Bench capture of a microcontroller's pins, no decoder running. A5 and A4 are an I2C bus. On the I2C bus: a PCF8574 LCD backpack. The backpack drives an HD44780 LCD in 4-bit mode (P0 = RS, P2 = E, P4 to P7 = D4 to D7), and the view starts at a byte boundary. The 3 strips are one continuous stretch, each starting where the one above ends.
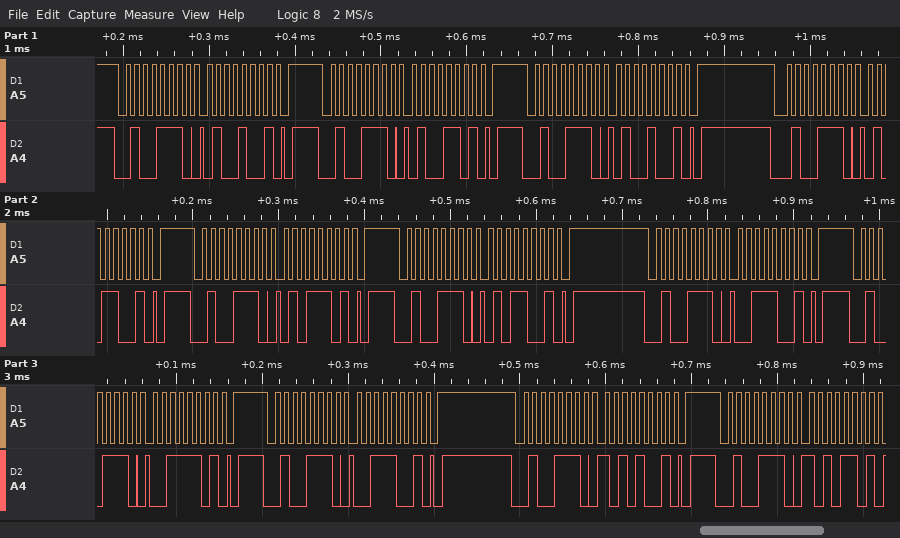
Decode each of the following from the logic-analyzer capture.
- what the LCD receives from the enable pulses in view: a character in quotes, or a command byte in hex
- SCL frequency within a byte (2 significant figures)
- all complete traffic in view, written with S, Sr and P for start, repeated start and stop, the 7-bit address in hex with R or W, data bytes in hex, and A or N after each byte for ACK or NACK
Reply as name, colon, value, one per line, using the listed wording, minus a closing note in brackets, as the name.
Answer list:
what the LCD receives from the enable pulses in view: a character in quotes, or a command byte in hex: 'E'
SCL frequency within a byte: 100 kHz
all complete traffic in view, written with S, Sr and P for start, repeated start and stop, the 7-bit address in hex with R or W, data bytes in hex, and A or N after each byte for ACK or NACK: S 27W A 49 A P S 27W A 4D A P S 27W A 49 A P S 27W A 59 A P S 27W A 5D A P S 27W A 59 A P S 27W A 39 A P S 27W A 3D A P S 27W A 39 A P S 27W A A9 A P S 27W A AD A
